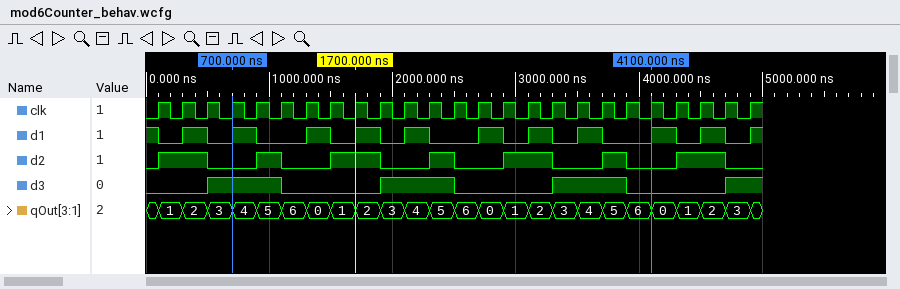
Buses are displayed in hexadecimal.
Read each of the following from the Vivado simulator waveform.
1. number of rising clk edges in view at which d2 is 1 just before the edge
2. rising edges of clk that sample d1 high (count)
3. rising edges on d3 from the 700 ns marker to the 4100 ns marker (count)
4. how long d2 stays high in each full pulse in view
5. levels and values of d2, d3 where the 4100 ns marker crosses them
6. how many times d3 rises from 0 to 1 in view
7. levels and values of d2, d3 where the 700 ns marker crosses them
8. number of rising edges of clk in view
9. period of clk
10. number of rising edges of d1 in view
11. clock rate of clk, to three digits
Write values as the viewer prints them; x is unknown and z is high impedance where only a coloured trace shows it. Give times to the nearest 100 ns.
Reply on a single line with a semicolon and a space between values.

11; 11; 2; 400 ns, 200 ns, 400 ns, 200 ns, 400 ns, 200 ns, 400 ns; d2=0, d3=0; 4; d2=0, d3=1; 25; 200 ns; 11; 5.00 MHz
